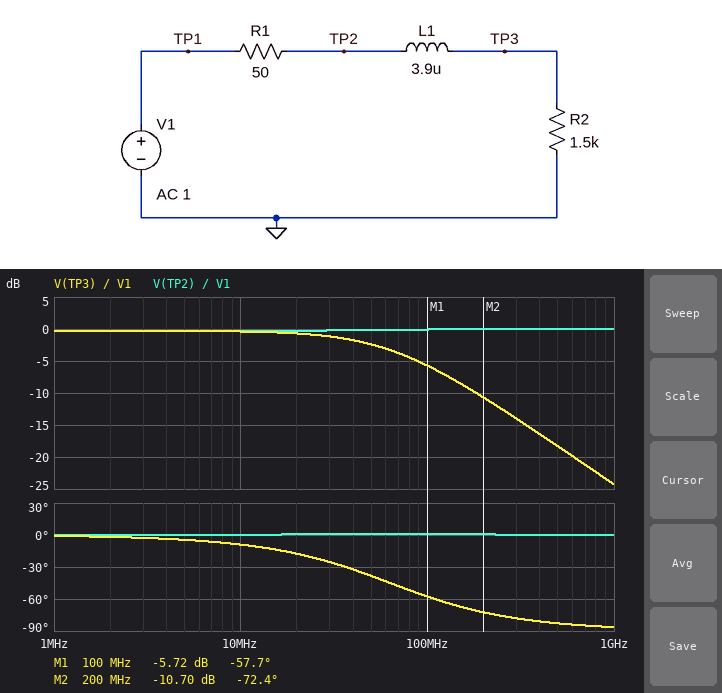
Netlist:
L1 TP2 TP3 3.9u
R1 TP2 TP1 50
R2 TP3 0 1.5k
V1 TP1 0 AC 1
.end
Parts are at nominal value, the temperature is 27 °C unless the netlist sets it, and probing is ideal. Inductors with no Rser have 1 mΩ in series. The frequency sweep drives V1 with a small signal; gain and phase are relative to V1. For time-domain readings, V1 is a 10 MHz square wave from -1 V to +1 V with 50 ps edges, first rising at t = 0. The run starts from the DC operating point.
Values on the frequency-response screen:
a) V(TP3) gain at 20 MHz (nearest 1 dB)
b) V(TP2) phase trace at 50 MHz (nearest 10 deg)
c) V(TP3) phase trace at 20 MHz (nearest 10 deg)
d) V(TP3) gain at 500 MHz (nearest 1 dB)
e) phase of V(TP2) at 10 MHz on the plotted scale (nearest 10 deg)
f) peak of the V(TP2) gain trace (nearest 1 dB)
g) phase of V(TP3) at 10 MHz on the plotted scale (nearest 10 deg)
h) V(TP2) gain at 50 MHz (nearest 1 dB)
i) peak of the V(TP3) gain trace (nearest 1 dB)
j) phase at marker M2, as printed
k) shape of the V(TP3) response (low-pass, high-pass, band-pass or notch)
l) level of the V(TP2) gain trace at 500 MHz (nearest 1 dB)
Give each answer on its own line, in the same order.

-1 dB
0 deg
-20 deg
-18 dB
0 deg
0 dB
-10 deg
0 dB
0 dB
-72.4 deg
low-pass
0 dB
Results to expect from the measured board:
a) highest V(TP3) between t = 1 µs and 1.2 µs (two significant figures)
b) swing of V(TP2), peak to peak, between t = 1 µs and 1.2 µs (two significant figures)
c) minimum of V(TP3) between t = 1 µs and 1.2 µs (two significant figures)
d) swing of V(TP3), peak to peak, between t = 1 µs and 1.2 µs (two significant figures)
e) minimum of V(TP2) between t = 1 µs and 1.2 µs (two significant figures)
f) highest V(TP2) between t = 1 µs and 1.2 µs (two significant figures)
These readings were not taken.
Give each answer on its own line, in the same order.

970 mV
2.1 V
-970 mV
1.9 V
-1.0 V
1.0 V
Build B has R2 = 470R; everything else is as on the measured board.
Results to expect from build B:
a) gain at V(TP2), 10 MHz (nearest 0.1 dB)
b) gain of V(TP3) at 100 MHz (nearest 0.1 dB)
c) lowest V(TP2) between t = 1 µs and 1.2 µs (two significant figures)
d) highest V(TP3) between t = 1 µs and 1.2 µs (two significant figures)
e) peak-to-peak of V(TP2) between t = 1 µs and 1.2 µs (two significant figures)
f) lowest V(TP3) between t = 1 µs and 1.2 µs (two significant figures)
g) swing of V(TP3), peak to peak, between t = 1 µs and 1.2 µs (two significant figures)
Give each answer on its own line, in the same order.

-0.7 dB
-14.5 dB
-1.1 V
900 mV
2.2 V
-900 mV
1.8 V
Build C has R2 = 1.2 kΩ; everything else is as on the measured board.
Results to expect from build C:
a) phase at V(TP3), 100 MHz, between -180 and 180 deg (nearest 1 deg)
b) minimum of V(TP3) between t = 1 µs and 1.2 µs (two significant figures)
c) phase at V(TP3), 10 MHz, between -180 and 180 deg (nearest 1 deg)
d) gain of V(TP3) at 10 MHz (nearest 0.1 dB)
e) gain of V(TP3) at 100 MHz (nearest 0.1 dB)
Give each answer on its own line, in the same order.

-63 deg
-960 mV
-11 deg
-0.5 dB
-7.2 dB
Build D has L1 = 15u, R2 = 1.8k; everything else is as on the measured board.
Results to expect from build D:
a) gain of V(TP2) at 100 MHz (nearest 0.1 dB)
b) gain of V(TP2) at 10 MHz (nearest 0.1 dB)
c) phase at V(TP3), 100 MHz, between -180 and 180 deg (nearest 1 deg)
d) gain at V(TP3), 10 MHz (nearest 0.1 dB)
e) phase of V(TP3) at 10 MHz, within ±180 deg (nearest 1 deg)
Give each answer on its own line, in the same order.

0 dB
-0.2 dB
-79 deg
-1.2 dB
-27 deg
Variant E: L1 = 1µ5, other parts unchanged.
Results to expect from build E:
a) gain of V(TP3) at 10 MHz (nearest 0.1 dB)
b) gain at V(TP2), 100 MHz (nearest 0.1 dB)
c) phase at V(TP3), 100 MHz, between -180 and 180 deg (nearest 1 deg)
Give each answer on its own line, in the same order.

-0.3 dB
-0.2 dB
-31 deg
